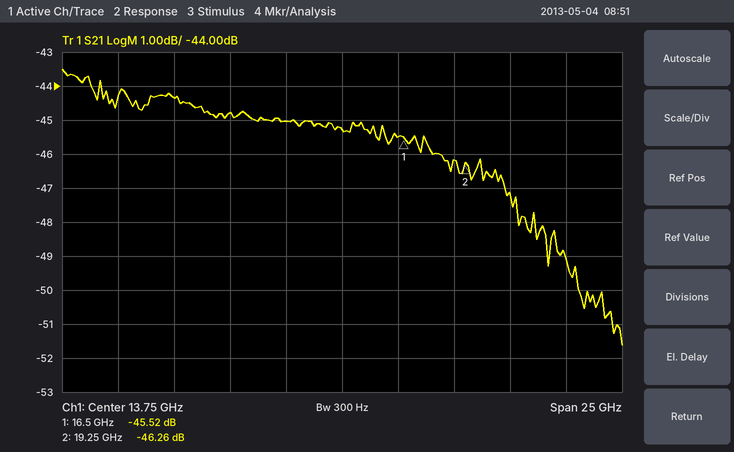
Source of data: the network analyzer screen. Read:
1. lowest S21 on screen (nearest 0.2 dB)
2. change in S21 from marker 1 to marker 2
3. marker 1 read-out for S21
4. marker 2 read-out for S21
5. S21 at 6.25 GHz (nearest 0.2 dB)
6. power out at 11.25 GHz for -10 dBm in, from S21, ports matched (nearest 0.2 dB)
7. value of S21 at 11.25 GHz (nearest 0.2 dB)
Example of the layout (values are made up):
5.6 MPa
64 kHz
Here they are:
-51.6 dB
-0.74 dB
-45.52 dB
-46.26 dB
-44.4 dB
-55.0 dBm
-45.0 dB
